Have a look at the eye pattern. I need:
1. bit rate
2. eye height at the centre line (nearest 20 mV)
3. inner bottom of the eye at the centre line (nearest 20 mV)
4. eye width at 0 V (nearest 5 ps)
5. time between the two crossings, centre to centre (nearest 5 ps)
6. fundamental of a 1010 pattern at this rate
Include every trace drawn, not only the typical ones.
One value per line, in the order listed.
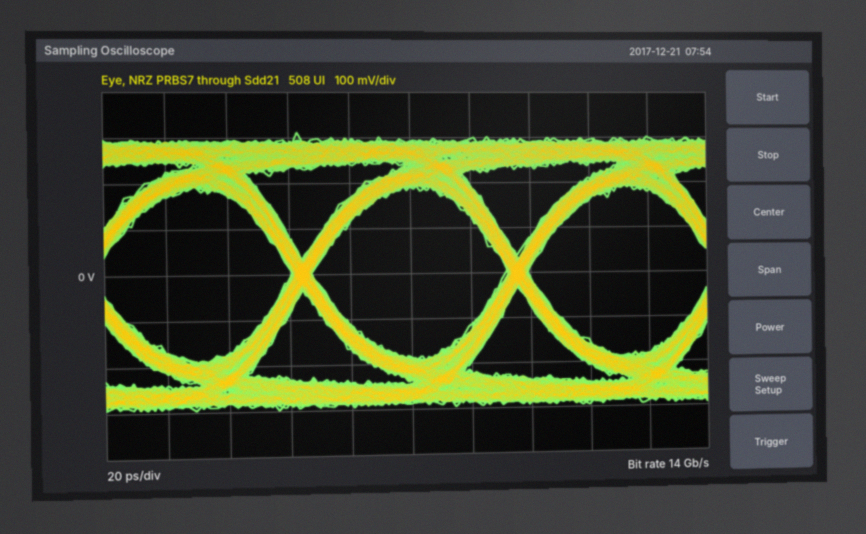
14 Gb/s
380 mV
-180 mV
65 ps
70 ps
7 GHz
